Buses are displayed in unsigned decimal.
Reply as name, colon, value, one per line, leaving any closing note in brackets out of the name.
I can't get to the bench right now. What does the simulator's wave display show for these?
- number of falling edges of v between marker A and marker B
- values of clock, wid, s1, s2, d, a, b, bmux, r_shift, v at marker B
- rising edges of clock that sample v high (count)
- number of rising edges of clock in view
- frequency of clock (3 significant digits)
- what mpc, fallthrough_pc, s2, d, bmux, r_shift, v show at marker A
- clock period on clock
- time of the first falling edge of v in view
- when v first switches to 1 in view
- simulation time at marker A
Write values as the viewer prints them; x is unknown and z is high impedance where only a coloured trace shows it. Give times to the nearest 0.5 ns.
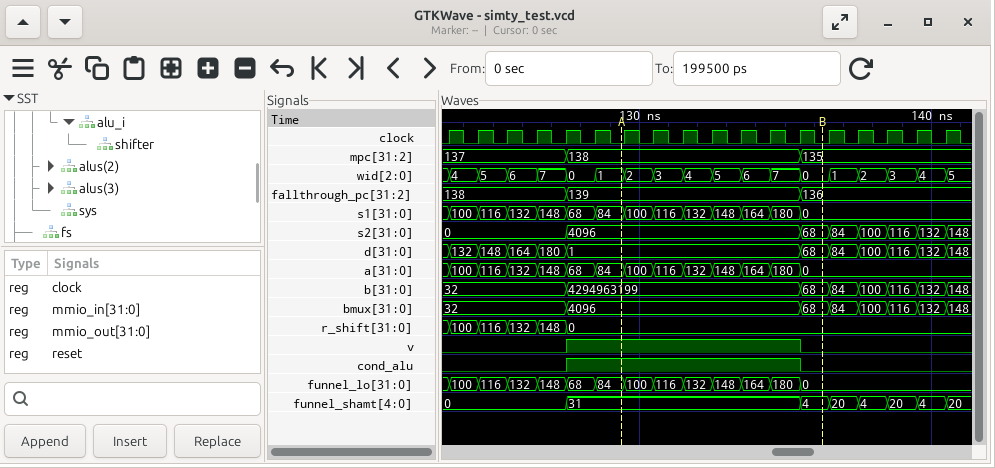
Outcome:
number of falling edges of v between marker A and marker B: 1
values of clock, wid, s1, s2, d, a, b, bmux, r_shift, v at marker B: clock=0, wid=0, s1=0, s2=68, d=68, a=0, b=68, bmux=68, r_shift=0, v=0
rising edges of clock that sample v high: 8
number of rising edges of clock in view: 18
frequency of clock: 1.00 GHz
what mpc, fallthrough_pc, s2, d, bmux, r_shift, v show at marker A: mpc=138, fallthrough_pc=139, s2=4096, d=1, bmux=4096, r_shift=0, v=1
clock period on clock: 1 ns
time of the first falling edge of v in view: 135.5 ns
when v first switches to 1 in view: 127.5 ns
simulation time at marker A: 129.5 ns
